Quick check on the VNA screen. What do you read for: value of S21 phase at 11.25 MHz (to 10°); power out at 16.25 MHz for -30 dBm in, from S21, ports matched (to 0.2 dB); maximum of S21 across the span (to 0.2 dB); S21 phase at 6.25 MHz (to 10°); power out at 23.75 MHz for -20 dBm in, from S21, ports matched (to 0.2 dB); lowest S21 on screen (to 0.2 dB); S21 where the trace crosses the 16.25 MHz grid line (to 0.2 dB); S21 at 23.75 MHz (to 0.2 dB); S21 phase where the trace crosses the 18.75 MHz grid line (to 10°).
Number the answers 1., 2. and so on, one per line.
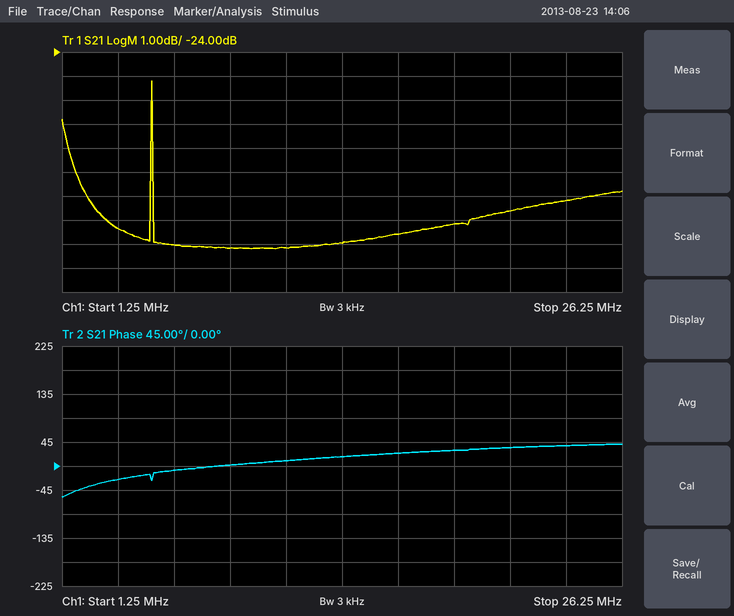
1. 10°
2. -61.6 dBm
3. -25.2 dB
4. -10°
5. -50.2 dBm
6. -32.2 dB
7. -31.6 dB
8. -30.2 dB
9. 30°
